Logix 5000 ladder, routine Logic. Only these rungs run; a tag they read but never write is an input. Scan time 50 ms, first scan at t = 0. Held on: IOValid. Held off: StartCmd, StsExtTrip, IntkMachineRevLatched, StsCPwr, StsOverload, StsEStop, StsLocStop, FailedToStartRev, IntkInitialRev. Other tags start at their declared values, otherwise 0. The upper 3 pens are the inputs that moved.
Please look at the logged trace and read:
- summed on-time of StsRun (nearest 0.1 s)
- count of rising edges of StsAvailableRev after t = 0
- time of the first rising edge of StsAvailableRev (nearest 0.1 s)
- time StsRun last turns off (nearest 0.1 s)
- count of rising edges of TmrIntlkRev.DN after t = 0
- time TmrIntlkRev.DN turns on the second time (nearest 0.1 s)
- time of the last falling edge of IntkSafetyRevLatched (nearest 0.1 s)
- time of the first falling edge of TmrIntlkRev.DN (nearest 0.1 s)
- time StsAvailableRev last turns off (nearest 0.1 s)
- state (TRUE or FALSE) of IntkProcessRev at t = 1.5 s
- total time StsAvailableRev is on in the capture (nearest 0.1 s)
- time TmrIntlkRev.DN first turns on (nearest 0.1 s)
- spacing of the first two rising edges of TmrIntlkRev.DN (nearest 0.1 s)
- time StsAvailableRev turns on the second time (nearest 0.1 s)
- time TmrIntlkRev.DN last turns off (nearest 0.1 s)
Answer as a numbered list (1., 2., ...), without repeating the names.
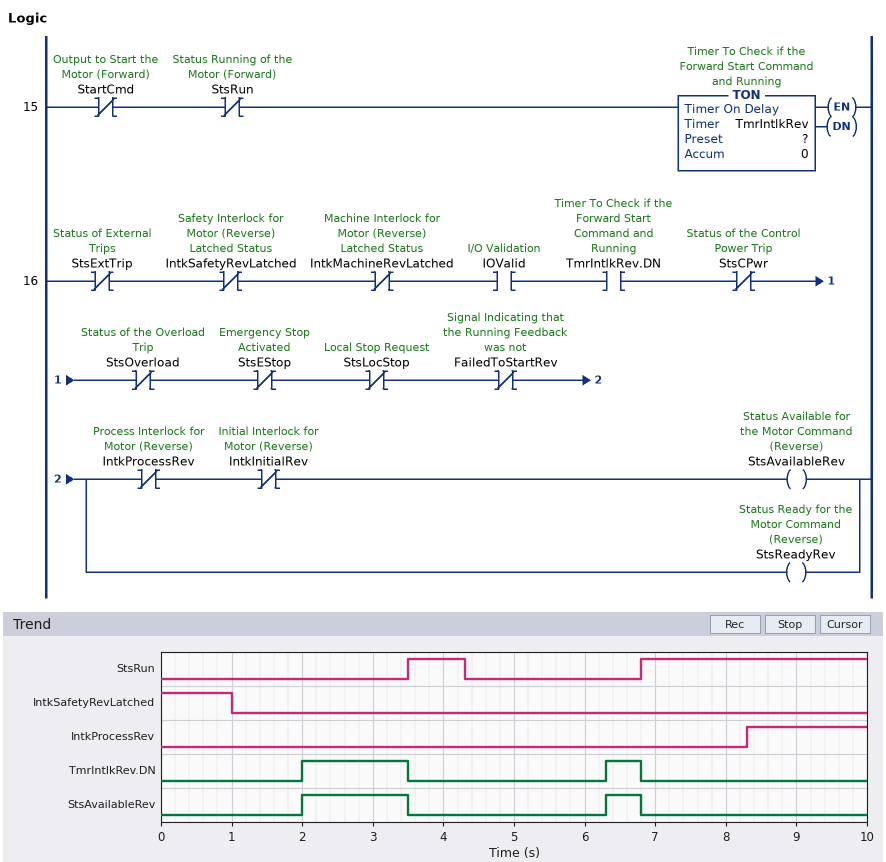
1. 4.0 s
2. 2
3. 2.0 s
4. 4.3 s
5. 2
6. 6.3 s
7. 1.0 s
8. 3.5 s
9. 6.8 s
10. FALSE
11. 2.0 s
12. 2.0 s
13. 4.3 s
14. 6.3 s
15. 6.8 s
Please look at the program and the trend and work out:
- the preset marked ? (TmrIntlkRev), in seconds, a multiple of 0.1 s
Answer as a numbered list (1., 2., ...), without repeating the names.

1. 2.0 s
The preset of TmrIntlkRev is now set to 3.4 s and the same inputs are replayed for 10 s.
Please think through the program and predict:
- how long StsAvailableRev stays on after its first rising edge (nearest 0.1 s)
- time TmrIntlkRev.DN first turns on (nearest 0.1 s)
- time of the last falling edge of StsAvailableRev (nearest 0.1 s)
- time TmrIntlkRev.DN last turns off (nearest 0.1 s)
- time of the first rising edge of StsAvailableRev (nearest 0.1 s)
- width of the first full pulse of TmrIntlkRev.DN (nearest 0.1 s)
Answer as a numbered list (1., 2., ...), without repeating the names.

1. 0.1 s
2. 3.4 s
3. 3.5 s
4. 3.5 s
5. 3.4 s
6. 0.1 s
